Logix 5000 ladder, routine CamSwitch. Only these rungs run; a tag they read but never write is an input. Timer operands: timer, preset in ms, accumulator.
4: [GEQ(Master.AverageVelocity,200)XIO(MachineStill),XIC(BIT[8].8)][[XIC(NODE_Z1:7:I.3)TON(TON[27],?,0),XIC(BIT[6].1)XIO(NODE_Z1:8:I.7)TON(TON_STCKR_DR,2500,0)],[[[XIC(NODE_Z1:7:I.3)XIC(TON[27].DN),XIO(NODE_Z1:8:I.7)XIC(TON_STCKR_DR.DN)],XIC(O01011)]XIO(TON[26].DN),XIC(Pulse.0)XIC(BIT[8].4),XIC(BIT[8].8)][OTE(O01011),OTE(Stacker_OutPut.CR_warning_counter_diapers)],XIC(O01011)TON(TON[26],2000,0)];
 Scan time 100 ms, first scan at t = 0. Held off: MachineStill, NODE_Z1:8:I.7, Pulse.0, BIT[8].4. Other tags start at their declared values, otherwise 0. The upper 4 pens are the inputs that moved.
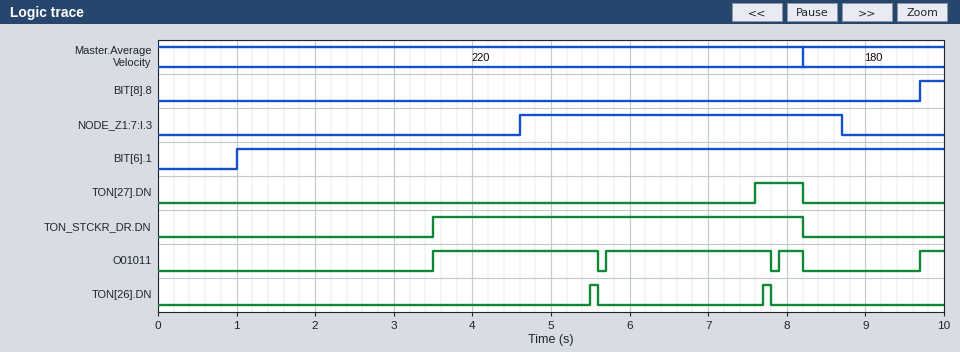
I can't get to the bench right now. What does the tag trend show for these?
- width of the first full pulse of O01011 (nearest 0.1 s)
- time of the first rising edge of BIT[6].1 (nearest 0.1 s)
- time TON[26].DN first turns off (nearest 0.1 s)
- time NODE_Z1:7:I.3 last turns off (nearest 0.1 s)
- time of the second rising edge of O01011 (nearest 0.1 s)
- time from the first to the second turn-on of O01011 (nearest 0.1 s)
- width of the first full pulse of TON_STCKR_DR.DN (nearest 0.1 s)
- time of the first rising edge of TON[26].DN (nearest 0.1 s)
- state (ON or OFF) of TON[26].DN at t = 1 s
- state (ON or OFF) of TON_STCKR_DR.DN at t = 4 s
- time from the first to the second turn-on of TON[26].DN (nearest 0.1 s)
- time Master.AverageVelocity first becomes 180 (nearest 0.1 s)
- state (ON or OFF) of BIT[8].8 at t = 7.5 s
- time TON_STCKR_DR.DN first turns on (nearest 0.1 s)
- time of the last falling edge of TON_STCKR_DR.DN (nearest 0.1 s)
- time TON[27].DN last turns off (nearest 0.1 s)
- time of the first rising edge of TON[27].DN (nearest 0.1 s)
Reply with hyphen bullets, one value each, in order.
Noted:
- 2.1 s
- 1.0 s
- 5.6 s
- 8.7 s
- 5.7 s
- 2.2 s
- 4.7 s
- 5.5 s
- OFF
- ON
- 2.2 s
- 8.2 s
- OFF
- 3.5 s
- 8.2 s
- 8.2 s
- 7.6 s
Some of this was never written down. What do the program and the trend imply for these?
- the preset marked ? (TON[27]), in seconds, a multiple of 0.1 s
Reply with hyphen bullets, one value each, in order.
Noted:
- 3.0 s
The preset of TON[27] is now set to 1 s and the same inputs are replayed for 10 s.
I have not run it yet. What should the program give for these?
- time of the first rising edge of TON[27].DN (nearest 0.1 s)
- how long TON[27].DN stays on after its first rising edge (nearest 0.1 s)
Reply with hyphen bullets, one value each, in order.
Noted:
- 5.6 s
- 2.6 s
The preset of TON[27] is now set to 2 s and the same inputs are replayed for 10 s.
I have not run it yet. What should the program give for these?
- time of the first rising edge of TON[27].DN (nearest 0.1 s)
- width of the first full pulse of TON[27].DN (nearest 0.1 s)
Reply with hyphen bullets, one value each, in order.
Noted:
- 6.6 s
- 1.6 s
